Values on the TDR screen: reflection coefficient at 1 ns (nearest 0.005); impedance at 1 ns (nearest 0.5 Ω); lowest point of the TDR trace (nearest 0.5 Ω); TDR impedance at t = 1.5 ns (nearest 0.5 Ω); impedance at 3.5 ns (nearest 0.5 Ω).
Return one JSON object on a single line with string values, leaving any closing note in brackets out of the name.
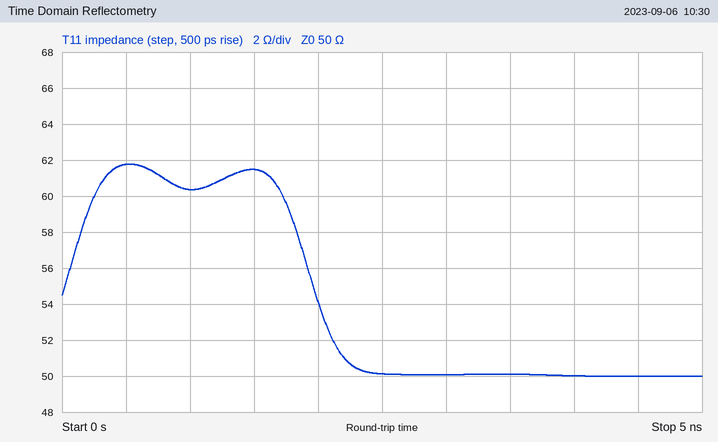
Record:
{"reflection coefficient at 1 ns": "+0.095", "impedance at 1 ns": "60.5 Ω", "lowest point of the TDR trace": "50.0 Ω", "TDR impedance at t = 1.5 ns": "61.5 Ω", "impedance at 3.5 ns": "50.0 Ω"}
